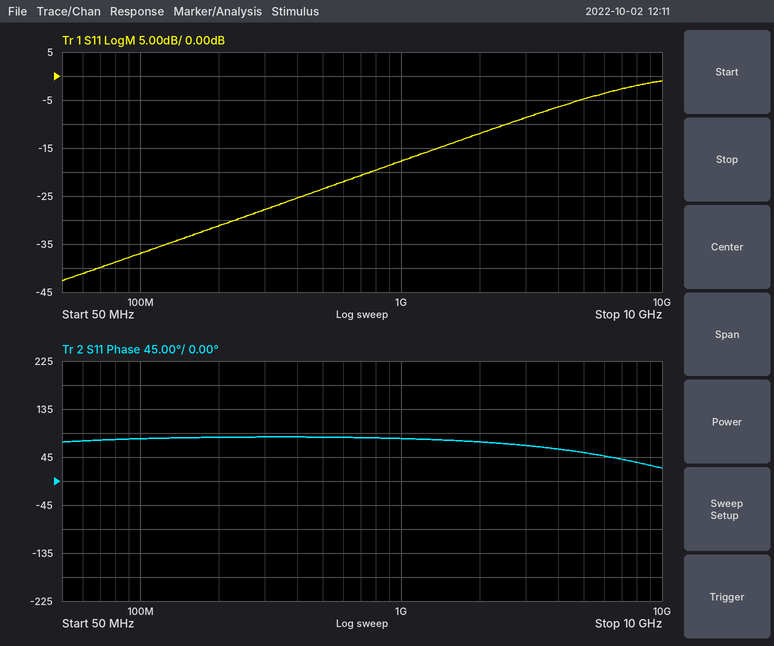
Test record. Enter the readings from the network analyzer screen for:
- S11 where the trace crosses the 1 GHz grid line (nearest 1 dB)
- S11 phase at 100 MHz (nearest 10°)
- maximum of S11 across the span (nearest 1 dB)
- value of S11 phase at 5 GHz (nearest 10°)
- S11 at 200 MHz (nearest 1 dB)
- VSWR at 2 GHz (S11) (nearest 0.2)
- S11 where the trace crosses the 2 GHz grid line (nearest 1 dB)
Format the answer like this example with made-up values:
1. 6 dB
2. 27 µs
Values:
1. -18 dB
2. 80°
3. -1 dB
4. 50°
5. -31 dB
6. 1.6
7. -12 dB
